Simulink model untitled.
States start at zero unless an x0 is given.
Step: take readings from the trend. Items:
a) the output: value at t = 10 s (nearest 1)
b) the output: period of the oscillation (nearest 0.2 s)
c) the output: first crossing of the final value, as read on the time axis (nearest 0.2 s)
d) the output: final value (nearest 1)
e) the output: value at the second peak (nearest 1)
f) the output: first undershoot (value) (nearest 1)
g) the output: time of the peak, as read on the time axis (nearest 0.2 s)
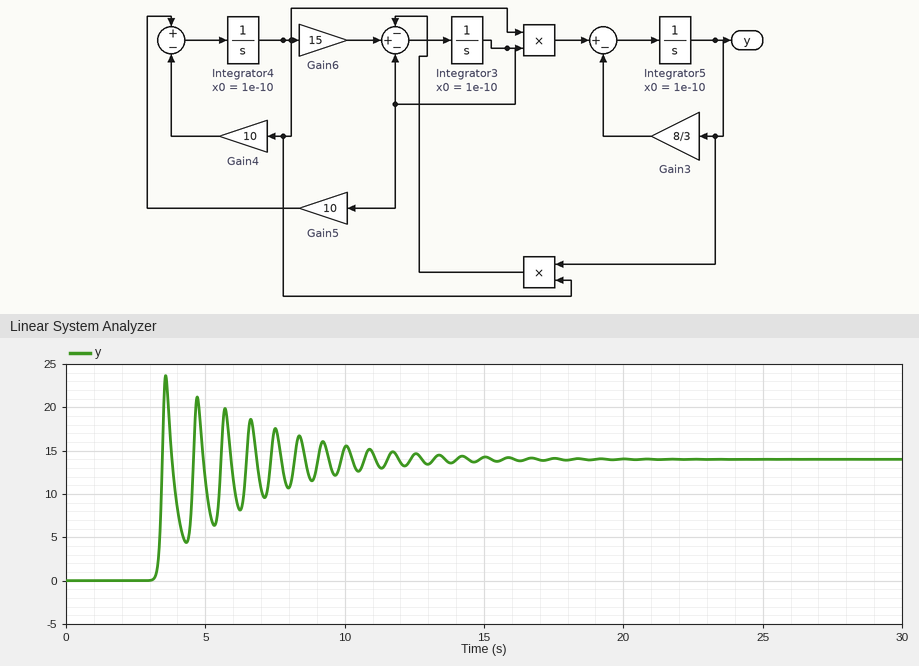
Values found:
15
1.2 s
3.4 s
14
21
4
3.6 s
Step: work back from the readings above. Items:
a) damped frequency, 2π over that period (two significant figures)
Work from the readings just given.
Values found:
5.2 rad/s
